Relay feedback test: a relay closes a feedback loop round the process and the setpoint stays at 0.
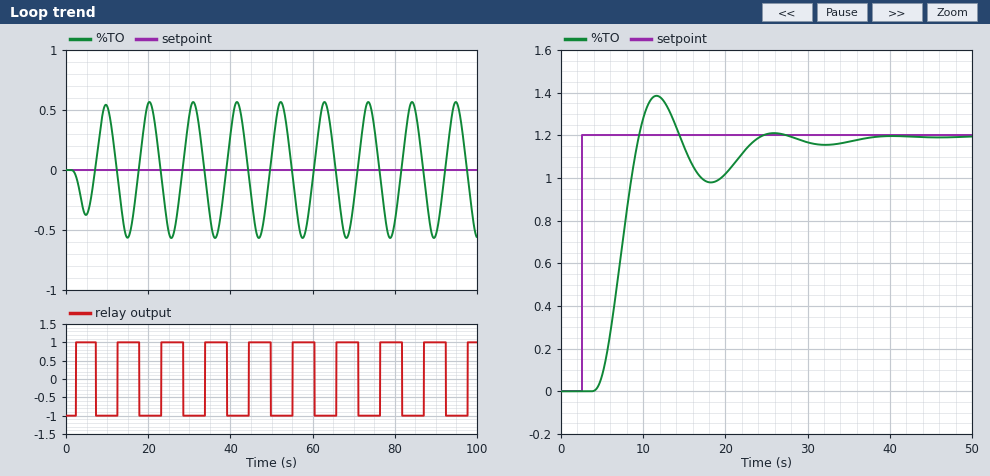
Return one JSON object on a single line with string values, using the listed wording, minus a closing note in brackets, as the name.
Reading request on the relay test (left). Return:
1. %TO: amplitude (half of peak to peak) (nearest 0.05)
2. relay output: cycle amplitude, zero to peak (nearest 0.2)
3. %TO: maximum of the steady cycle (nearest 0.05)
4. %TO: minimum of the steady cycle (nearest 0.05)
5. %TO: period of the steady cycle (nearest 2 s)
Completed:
{"%TO: amplitude (half of peak to peak)": "0.55", "relay output: cycle amplitude, zero to peak": "1.0", "%TO: maximum of the steady cycle": "0.55", "%TO: minimum of the steady cycle": "-0.55", "%TO: period of the steady cycle": "10 s"}
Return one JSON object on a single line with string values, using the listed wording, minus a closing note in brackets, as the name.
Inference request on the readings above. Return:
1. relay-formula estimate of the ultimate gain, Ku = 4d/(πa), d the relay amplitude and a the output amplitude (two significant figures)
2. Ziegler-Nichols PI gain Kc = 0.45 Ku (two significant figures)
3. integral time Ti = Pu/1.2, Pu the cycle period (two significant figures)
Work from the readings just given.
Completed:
{"relay-formula estimate of the ultimate gain, Ku = 4d/(πa), d the relay amplitude and a the output amplitude": "2.3", "Ziegler-Nichols PI gain Kc = 0.45 Ku": "1.0", "integral time Ti = Pu/1.2, Pu the cycle period": "8.3 s"}
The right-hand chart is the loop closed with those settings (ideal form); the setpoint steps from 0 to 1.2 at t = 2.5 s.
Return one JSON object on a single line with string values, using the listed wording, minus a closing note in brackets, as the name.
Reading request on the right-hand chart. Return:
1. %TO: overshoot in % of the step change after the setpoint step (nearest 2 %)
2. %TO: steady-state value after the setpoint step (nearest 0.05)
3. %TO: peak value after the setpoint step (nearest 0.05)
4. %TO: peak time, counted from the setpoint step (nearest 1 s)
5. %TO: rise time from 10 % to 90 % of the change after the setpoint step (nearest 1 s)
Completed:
{"%TO: overshoot in % of the step change after the setpoint step": "16 %", "%TO: steady-state value after the setpoint step": "1.20", "%TO: peak value after the setpoint step": "1.40", "%TO: peak time, counted from the setpoint step": "9 s", "%TO: rise time from 10 % to 90 % of the change after the setpoint step": "4 s"}
